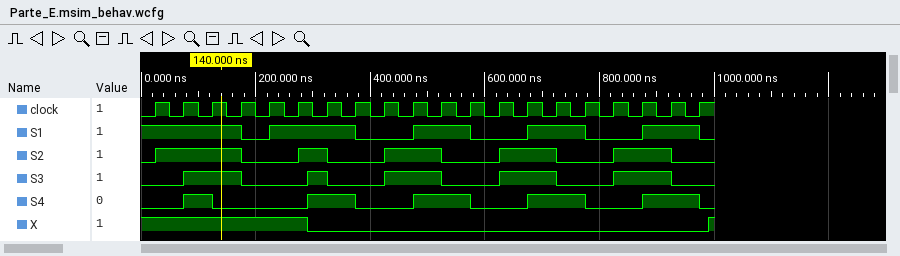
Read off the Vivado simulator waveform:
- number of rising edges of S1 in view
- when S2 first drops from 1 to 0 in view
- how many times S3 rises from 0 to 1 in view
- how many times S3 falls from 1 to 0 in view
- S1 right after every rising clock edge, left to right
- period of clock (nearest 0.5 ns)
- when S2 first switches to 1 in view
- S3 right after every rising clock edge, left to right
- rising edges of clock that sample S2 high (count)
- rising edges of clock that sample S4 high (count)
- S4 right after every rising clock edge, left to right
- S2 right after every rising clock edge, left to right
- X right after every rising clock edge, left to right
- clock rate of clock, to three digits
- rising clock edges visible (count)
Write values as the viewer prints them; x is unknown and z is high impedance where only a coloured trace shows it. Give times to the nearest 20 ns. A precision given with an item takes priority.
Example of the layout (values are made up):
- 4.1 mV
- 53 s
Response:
- 4
- 180 ns
- 5
- 5
- 1 1 1 0 1 1 1 0 0 1 1 0 0 1 1 0 0 1 1 0
- 50 ns
- 20 ns
- 0 1 1 0 0 0 0 0 1 1 0 0 1 1 0 0 1 1 0 0
- 10
- 9
- 0 1 0 0 0 0 1 0 0 1 1 0 0 1 1 0 0 1 1 0
- 1 1 1 0 0 1 0 0 1 1 0 0 1 1 0 0 1 1 0 0
- 1 1 1 1 1 1 0 0 0 0 0 0 0 0 0 0 0 0 0 0
- 20.0 MHz
- 20
